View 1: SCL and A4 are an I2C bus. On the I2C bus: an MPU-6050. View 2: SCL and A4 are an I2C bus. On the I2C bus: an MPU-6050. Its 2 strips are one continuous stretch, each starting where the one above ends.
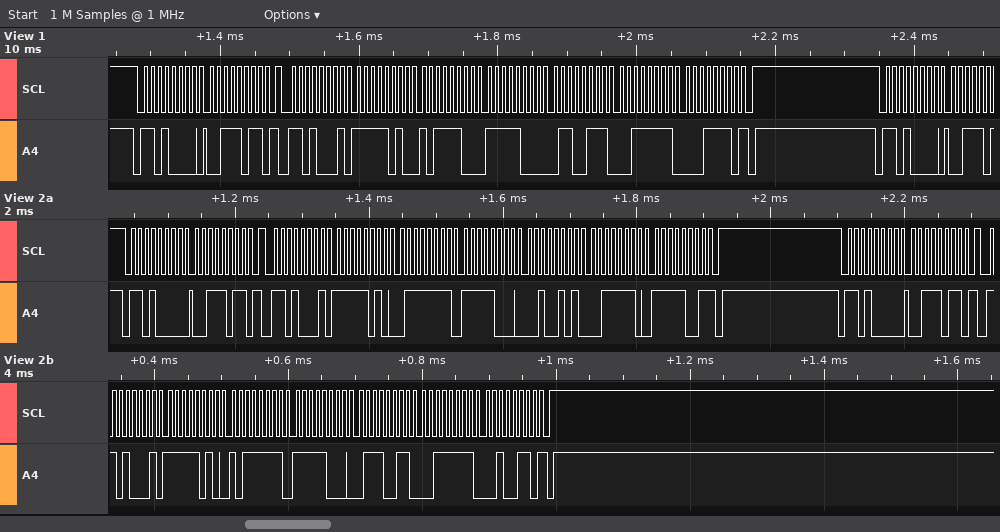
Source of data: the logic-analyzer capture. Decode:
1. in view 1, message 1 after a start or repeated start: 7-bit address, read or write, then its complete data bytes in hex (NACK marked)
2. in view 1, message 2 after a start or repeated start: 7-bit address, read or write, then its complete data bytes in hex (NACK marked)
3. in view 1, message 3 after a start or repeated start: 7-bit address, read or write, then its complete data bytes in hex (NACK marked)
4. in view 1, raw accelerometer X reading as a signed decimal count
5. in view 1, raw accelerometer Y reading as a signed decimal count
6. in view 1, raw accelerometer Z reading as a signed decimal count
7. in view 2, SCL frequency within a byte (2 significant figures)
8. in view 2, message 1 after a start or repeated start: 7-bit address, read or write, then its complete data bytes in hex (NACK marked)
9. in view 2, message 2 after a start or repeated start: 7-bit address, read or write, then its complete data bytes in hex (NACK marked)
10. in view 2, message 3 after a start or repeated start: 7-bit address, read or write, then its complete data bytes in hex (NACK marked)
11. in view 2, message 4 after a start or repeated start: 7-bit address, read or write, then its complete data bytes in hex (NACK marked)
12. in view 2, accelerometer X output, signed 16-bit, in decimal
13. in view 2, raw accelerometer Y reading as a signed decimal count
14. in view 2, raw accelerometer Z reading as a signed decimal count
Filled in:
0x68 write: 3B
0x68 read: FA BC F8 67 3F 1E NACK
0x68 write
-1348
-1945
16158
100 kHz
0x68 write: 3B
0x68 read: FA 7F F8 25 3E F9 NACK
0x68 write: 3B
0x68 read: FA BF F8 73 3F 26 NACK
-1409
-2011
16121
